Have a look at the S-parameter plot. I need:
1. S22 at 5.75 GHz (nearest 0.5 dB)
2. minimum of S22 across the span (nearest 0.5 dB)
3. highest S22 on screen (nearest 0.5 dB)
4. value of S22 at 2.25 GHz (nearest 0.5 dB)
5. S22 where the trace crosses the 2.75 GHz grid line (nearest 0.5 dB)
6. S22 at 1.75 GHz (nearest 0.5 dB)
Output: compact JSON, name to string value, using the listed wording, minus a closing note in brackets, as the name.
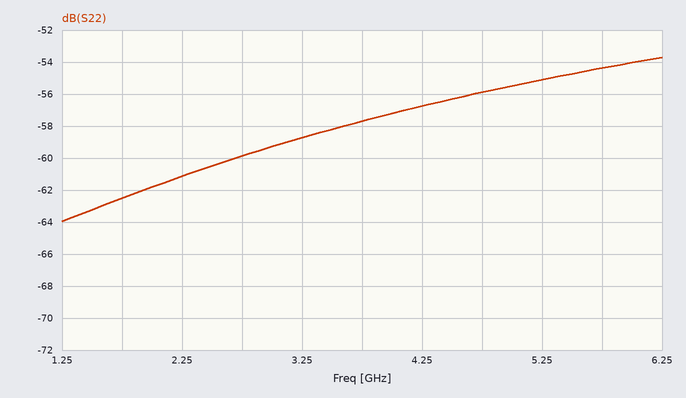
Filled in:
{"S22 at 5.75 GHz": "-54.5 dB", "minimum of S22 across the span": "-64.0 dB", "highest S22 on screen": "-53.5 dB", "value of S22 at 2.25 GHz": "-61.0 dB", "S22 where the trace crosses the 2.75 GHz grid line": "-60.0 dB", "S22 at 1.75 GHz": "-62.5 dB"}
